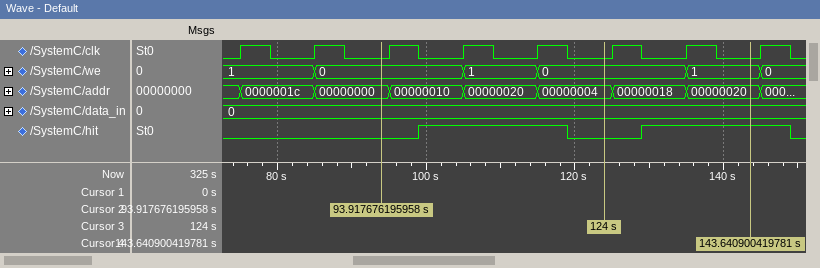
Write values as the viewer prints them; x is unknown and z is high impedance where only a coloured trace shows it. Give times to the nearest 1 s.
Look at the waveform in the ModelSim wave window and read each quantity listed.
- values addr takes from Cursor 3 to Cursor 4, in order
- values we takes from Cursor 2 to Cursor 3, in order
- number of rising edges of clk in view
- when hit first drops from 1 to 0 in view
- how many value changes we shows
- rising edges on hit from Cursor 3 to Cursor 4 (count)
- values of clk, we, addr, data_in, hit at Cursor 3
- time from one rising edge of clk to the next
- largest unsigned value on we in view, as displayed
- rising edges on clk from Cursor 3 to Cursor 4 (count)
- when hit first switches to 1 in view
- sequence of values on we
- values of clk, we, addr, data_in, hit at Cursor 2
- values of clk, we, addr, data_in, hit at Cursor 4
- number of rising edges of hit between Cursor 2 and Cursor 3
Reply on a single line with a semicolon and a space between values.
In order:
00000004, 00000018, 00000020; 0, 1, 0; 8; 119 s; 5; 1; clk=0, we=0, addr=00000004, data_in=0, hit=0; 10 s; 1; 2; 99 s; 1, 0, 1, 0, 1, 0; clk=0, we=0, addr=00000000, data_in=0, hit=0; clk=0, we=1, addr=00000020, data_in=0, hit=1; 1
